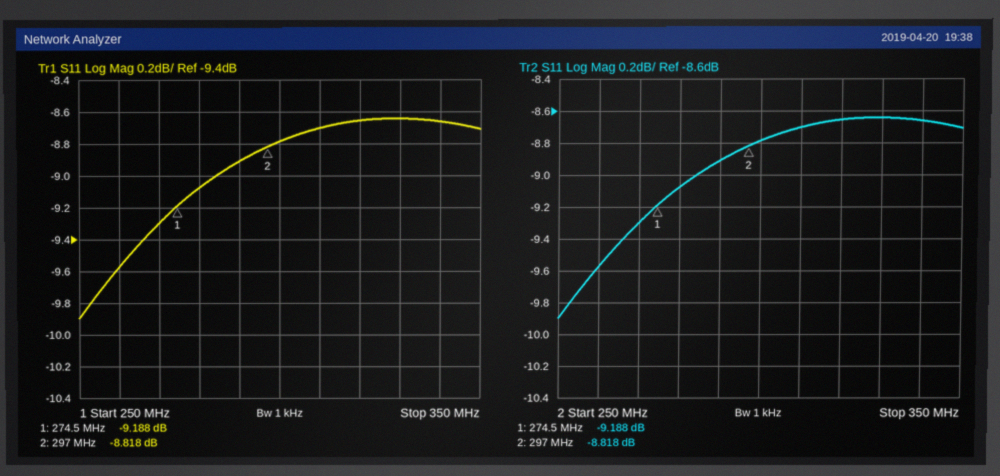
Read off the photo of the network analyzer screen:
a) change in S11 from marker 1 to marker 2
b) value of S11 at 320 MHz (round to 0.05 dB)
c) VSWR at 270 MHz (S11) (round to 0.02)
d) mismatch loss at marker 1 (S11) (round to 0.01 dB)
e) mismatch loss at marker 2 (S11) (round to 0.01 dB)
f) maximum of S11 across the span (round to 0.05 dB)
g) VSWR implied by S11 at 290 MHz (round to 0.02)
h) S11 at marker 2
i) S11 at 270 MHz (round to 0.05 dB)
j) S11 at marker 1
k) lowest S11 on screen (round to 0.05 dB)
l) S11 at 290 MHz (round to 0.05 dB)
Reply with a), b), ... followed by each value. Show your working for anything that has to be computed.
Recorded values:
a) -8.818 − (-9.188) = 0.370 dB
b) -8.65 dB
c) |Γ| = 10^(-9.3/20) = 0.3428; VSWR = (1 + 0.3428)/(1 − 0.3428) ≈ 2.04
d) −10 log10(1 − 10^(-9.188/10)) ≈ 0.56 dB
e) −10 log10(1 − 10^(-8.818/10)) ≈ 0.61 dB
f) -8.65 dB
g) |Γ| = 10^(-8.9/20) = 0.3589; VSWR = (1 + 0.3589)/(1 − 0.3589) ≈ 2.12
h) -8.818 dB
i) -9.30 dB
j) -9.188 dB
k) -9.90 dB
l) -8.90 dB
